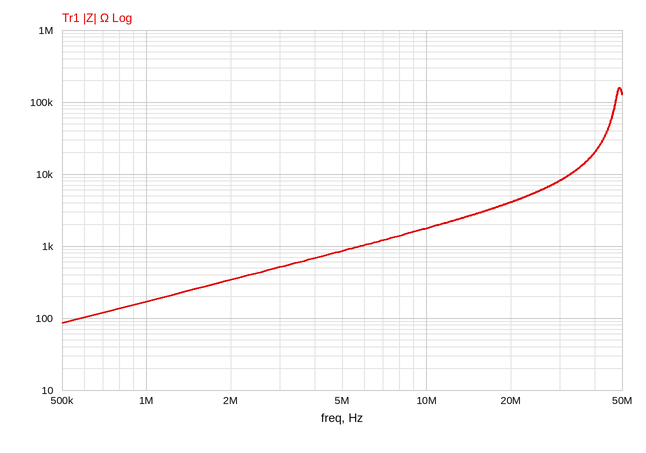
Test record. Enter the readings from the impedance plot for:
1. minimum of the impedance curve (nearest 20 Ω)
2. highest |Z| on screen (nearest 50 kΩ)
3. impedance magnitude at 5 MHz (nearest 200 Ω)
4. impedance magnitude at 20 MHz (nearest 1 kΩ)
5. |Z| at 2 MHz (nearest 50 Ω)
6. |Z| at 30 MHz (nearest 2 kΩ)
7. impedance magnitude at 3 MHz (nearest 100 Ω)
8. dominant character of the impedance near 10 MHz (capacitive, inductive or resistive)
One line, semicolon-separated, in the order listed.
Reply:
80 Ω; 150 kΩ; 800 Ω; 4 kΩ; 350 Ω; 8 kΩ; 500 Ω; inductive
